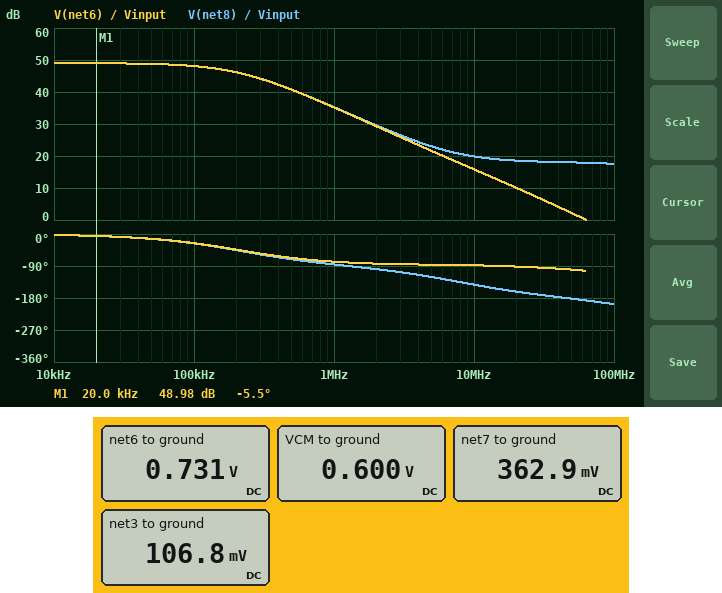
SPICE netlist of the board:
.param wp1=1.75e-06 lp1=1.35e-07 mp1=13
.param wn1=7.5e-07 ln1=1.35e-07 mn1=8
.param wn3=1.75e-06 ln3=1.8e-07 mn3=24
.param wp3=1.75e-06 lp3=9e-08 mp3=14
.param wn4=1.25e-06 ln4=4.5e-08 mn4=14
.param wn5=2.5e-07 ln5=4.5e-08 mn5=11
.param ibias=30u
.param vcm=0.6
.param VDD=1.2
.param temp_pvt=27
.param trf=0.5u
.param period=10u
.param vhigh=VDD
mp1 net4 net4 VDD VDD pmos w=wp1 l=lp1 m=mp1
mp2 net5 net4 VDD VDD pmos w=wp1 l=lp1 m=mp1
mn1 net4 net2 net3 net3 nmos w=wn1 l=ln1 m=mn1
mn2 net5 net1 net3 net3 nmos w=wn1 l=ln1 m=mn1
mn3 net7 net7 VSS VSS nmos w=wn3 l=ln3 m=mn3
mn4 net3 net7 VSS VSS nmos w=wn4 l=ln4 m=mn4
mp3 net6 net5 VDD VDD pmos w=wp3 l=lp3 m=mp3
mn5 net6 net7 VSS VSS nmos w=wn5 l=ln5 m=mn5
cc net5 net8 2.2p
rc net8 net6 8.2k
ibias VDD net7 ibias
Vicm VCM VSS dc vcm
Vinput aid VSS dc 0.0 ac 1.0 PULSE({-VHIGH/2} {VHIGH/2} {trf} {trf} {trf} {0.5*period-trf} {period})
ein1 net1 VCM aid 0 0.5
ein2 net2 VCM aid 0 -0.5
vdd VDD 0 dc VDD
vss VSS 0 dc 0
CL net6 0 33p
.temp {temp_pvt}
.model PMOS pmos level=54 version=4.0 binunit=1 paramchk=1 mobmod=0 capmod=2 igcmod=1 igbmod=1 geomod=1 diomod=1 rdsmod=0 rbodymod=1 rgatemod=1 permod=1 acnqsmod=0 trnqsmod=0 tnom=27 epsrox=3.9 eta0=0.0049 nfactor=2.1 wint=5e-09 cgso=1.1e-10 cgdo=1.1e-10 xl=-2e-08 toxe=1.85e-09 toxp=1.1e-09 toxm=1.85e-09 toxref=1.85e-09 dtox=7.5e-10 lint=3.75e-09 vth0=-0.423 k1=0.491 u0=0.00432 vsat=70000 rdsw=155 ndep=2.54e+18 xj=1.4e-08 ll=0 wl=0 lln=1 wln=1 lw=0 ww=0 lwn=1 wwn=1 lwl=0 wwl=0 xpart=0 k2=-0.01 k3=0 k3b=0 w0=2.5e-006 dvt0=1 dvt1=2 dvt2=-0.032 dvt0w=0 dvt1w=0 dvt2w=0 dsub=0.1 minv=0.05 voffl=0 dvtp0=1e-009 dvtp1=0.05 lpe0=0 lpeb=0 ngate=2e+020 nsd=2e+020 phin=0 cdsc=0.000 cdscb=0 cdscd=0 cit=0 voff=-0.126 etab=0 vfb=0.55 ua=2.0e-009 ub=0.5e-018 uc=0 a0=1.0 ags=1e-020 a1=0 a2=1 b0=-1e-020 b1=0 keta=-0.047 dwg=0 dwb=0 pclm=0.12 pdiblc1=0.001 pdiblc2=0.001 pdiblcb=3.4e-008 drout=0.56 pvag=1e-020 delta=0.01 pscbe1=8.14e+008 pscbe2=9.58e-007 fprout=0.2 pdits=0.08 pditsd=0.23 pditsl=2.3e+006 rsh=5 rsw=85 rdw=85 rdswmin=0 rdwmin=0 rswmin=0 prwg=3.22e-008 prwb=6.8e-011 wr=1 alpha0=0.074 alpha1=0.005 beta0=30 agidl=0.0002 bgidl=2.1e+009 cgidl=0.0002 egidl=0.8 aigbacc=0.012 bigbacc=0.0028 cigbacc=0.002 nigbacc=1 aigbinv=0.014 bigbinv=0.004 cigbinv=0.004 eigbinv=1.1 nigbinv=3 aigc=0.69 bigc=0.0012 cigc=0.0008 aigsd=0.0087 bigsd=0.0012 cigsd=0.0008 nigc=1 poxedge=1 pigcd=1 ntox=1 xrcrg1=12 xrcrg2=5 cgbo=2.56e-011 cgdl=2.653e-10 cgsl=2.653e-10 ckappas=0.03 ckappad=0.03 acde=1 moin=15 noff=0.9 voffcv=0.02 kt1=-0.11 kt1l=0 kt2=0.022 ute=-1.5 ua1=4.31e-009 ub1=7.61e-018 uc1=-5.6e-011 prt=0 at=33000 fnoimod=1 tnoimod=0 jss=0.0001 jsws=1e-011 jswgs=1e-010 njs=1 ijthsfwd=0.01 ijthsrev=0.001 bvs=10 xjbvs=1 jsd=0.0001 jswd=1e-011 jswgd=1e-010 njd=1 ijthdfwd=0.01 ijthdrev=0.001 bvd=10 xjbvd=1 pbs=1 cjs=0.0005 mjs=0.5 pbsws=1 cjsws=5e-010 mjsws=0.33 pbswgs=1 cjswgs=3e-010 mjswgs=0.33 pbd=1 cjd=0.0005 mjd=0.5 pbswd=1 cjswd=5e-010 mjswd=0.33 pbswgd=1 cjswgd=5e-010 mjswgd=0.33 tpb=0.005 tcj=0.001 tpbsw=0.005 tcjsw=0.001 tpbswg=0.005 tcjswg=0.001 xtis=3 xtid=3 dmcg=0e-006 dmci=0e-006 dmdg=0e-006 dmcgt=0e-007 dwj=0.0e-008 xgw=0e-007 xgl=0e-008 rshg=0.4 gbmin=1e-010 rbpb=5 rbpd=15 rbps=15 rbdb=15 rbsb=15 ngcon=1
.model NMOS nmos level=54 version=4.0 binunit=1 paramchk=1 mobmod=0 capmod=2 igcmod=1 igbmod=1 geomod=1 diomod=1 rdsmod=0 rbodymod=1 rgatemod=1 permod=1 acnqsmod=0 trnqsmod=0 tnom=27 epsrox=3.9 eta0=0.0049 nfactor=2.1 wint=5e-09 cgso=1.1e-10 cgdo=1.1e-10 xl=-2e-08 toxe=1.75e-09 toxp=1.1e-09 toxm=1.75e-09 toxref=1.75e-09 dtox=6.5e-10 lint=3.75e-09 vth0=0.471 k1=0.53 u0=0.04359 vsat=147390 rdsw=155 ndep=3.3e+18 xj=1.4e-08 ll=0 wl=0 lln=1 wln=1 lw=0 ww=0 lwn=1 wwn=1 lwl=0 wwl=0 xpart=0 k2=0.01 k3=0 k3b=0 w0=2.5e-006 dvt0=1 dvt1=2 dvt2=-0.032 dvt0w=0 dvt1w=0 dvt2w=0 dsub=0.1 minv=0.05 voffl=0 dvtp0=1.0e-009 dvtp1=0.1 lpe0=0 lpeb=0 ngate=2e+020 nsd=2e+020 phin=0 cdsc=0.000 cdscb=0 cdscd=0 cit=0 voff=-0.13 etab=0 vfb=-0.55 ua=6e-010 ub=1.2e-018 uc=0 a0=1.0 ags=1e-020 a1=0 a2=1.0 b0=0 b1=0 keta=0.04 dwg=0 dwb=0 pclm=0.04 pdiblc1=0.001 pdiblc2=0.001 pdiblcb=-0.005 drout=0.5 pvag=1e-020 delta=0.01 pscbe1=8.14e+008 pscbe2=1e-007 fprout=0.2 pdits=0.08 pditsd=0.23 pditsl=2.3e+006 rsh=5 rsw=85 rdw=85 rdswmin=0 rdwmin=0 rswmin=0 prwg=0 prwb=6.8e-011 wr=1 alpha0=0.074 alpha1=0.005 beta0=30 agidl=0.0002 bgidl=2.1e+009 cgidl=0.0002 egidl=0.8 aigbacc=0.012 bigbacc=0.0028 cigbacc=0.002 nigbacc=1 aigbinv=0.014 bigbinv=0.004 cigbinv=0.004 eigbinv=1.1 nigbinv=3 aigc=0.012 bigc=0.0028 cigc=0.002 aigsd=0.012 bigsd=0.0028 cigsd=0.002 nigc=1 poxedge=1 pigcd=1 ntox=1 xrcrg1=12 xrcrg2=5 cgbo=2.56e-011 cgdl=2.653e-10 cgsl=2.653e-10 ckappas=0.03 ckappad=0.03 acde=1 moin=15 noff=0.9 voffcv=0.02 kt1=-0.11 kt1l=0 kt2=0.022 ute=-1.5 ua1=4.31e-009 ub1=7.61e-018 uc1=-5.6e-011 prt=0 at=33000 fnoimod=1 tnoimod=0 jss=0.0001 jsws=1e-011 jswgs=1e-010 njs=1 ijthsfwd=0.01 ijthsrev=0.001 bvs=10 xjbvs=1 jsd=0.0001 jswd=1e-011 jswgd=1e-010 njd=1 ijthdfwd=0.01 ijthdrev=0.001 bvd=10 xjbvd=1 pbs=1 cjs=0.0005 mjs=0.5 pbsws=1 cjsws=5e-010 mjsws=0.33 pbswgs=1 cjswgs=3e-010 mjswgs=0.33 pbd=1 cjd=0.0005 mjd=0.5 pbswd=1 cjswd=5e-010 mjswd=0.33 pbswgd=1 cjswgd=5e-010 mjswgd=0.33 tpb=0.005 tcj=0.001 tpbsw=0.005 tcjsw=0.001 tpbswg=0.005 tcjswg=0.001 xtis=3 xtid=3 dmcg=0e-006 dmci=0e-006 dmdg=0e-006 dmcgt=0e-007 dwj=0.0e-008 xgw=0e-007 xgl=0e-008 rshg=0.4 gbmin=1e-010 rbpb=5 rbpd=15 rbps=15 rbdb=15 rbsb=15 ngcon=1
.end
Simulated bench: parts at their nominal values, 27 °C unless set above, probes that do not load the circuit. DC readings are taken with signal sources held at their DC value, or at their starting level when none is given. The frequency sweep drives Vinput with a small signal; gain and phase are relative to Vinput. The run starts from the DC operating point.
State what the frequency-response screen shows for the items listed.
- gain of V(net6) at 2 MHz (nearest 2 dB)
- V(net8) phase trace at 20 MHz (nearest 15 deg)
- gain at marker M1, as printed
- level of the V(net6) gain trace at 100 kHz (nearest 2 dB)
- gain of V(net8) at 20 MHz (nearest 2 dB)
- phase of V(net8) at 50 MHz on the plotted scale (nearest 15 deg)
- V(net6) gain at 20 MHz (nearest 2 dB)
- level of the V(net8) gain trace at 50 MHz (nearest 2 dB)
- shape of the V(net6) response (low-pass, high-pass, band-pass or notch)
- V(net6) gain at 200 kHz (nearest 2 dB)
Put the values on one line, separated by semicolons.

30 dB; -165 deg; 48.98 dB; 48 dB; 18 dB; -180 deg; 10 dB; 18 dB; low-pass; 46 dB
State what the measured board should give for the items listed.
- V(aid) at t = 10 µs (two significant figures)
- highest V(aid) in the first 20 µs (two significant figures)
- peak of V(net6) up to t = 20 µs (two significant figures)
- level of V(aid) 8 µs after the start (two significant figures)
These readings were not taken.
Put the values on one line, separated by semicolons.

-600 mV; 600 mV; 1.2 V; -600 mV
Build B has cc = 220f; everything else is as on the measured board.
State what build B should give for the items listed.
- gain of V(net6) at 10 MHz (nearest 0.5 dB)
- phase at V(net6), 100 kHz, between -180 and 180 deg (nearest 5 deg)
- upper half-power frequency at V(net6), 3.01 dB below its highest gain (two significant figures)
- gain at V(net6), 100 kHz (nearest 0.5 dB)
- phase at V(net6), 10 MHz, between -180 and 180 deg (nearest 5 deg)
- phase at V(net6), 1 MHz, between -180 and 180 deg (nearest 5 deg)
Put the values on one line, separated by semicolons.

28.0 dB; -5 deg; 1.1 MHz; 49.0 dB; -110 deg; -45 deg
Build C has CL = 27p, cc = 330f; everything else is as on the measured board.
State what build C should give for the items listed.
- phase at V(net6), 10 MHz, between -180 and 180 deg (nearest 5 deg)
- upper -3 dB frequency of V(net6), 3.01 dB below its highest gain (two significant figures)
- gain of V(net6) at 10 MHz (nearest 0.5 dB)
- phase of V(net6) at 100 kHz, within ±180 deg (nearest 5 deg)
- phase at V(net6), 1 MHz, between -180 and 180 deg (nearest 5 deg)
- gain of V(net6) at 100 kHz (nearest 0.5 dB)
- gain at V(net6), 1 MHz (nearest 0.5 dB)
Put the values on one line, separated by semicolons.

-110 deg; 940 kHz; 27.0 dB; -5 deg; -50 deg; 49.0 dB; 45.5 dB
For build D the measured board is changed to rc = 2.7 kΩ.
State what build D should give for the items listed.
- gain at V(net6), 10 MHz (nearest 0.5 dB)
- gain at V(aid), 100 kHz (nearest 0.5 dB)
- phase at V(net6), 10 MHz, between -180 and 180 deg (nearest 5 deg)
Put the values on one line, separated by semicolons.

13.5 dB; 0 dB; -115 deg
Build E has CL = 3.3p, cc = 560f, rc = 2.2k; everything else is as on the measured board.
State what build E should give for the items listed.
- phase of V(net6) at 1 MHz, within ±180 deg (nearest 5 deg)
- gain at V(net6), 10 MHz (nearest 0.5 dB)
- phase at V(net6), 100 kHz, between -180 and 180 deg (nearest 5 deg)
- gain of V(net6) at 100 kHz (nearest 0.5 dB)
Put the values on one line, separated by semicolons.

-50 deg; 27.5 dB; -5 deg; 49.0 dB
